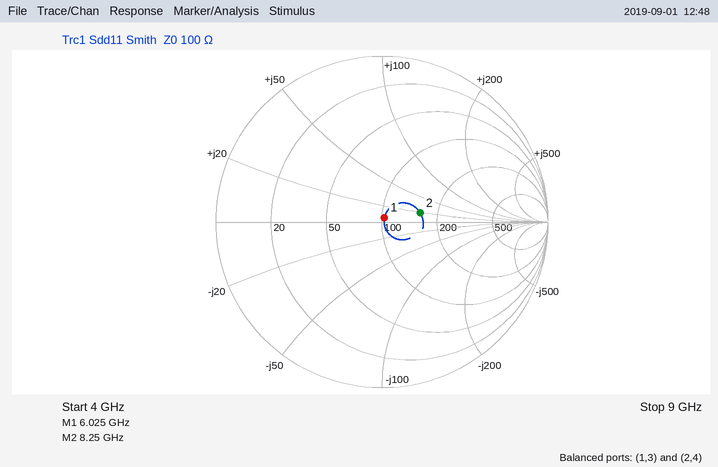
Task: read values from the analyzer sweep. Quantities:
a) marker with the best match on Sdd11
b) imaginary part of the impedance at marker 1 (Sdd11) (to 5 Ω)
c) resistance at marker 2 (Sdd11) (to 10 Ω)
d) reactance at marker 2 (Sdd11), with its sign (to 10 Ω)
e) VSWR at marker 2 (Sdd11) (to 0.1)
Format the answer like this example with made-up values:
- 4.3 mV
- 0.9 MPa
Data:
- marker 1
- +5 Ω
- 160 Ω
- +20 Ω
- 1.6
